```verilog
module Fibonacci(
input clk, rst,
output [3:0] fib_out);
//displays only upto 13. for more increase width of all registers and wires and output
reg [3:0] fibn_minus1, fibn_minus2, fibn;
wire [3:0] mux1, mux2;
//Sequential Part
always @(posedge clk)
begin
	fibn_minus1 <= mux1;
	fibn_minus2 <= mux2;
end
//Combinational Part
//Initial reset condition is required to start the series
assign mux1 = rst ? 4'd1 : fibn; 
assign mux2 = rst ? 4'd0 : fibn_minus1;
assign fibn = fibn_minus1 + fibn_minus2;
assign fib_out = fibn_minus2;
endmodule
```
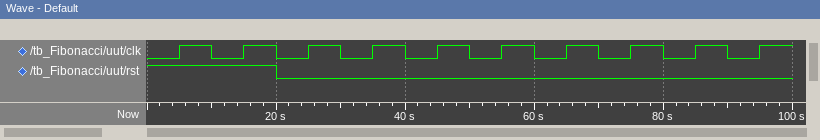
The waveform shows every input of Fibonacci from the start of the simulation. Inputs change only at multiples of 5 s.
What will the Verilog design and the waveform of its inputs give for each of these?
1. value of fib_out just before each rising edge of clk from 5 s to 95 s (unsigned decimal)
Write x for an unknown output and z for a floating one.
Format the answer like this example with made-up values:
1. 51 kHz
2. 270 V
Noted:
1. x, 0, 0, 1, 1, 2, 3, 5, 8, 13
